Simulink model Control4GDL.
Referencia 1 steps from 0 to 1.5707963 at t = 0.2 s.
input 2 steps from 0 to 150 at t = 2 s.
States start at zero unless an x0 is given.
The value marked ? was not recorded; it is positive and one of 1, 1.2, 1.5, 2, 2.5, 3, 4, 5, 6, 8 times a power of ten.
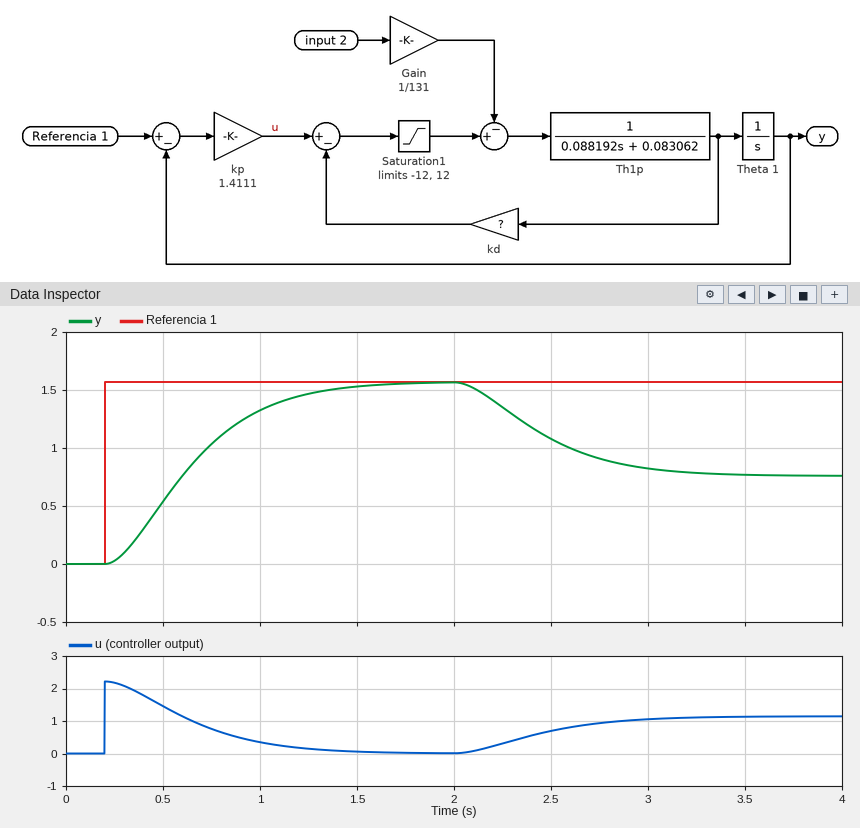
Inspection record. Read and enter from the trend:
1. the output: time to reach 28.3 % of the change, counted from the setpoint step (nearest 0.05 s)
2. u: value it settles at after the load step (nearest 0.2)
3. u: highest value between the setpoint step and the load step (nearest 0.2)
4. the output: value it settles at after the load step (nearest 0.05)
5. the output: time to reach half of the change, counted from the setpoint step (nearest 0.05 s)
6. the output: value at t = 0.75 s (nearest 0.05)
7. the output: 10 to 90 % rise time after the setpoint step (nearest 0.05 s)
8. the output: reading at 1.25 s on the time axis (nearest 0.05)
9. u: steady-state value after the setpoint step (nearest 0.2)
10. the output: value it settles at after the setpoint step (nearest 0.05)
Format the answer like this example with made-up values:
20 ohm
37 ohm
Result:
0.25 s
1.2
2.2
0.75
0.40 s
1.05
0.80 s
1.45
0.0
1.55
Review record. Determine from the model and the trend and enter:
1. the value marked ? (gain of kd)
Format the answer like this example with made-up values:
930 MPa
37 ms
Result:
0.6
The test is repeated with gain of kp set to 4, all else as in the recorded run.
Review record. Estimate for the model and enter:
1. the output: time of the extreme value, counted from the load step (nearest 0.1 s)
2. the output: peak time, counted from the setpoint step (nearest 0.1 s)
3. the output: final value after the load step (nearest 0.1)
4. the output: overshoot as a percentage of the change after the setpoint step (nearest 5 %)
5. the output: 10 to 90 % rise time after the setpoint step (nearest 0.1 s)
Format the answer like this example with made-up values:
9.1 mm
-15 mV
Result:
0.6 s
0.6 s
1.3
10 %
0.3 s
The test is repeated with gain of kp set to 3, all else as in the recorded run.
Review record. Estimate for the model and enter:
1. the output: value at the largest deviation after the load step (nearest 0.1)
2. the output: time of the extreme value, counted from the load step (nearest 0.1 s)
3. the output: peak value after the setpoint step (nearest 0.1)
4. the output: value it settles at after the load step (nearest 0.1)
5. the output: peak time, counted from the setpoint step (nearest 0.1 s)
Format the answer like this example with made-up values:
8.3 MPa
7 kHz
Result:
1.2
0.7 s
1.7
1.2
0.7 s
